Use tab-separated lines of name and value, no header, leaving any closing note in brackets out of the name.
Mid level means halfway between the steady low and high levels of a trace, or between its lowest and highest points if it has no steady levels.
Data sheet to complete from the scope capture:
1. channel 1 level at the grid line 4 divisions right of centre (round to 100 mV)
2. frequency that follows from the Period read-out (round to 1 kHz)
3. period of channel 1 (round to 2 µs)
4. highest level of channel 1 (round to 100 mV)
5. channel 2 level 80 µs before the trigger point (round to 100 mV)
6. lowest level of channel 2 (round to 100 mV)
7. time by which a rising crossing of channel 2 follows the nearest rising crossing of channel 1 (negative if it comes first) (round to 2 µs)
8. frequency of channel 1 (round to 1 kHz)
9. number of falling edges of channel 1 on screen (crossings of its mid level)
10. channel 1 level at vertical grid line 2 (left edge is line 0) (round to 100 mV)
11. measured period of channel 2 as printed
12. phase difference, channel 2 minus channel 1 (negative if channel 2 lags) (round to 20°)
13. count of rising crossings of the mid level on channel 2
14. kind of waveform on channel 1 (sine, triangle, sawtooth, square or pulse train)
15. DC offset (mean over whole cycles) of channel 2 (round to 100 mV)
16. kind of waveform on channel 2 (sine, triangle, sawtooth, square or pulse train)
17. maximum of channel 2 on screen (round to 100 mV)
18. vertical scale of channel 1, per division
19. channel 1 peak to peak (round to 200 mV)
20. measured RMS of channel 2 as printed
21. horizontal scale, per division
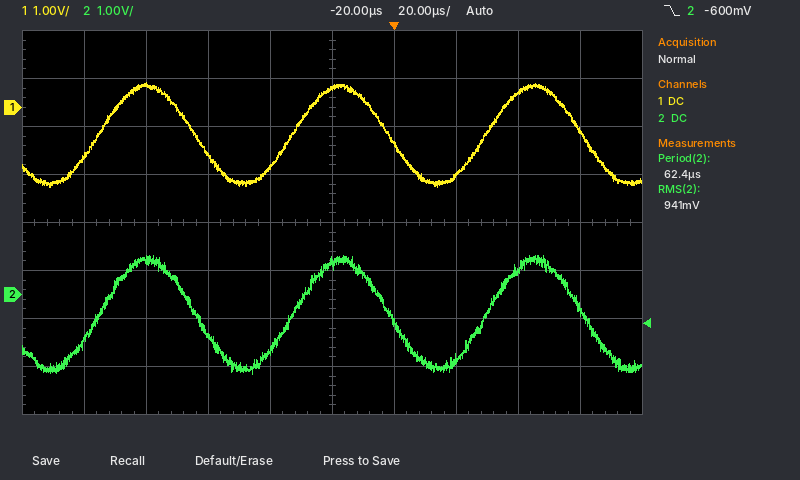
channel 1 level at the grid line 4 divisions right of centre	-500 mV
frequency that follows from the Period read-out	16 kHz
period of channel 1	62 µs
highest level of channel 1	500 mV
channel 2 level 80 µs before the trigger point	700 mV
lowest level of channel 2	-1.6 V
time by which a rising crossing of channel 2 follows the nearest rising crossing of channel 1 (negative if it comes first)	0 µs
frequency of channel 1	16 kHz
number of falling edges of channel 1 on screen	3
channel 1 level at vertical grid line 2 (left edge is line 0)	500 mV
measured period of channel 2 as printed	62.4 µs
phase difference, channel 2 minus channel 1 (negative if channel 2 lags)	0°
count of rising crossings of the mid level on channel 2	3
kind of waveform on channel 1	sine
DC offset (mean over whole cycles) of channel 2	-400 mV
kind of waveform on channel 2	sine
maximum of channel 2 on screen	800 mV
vertical scale of channel 1, per division	1 V
channel 1 peak to peak	2.2 V
measured RMS of channel 2 as printed	941 mV
horizontal scale, per division	20 µs
